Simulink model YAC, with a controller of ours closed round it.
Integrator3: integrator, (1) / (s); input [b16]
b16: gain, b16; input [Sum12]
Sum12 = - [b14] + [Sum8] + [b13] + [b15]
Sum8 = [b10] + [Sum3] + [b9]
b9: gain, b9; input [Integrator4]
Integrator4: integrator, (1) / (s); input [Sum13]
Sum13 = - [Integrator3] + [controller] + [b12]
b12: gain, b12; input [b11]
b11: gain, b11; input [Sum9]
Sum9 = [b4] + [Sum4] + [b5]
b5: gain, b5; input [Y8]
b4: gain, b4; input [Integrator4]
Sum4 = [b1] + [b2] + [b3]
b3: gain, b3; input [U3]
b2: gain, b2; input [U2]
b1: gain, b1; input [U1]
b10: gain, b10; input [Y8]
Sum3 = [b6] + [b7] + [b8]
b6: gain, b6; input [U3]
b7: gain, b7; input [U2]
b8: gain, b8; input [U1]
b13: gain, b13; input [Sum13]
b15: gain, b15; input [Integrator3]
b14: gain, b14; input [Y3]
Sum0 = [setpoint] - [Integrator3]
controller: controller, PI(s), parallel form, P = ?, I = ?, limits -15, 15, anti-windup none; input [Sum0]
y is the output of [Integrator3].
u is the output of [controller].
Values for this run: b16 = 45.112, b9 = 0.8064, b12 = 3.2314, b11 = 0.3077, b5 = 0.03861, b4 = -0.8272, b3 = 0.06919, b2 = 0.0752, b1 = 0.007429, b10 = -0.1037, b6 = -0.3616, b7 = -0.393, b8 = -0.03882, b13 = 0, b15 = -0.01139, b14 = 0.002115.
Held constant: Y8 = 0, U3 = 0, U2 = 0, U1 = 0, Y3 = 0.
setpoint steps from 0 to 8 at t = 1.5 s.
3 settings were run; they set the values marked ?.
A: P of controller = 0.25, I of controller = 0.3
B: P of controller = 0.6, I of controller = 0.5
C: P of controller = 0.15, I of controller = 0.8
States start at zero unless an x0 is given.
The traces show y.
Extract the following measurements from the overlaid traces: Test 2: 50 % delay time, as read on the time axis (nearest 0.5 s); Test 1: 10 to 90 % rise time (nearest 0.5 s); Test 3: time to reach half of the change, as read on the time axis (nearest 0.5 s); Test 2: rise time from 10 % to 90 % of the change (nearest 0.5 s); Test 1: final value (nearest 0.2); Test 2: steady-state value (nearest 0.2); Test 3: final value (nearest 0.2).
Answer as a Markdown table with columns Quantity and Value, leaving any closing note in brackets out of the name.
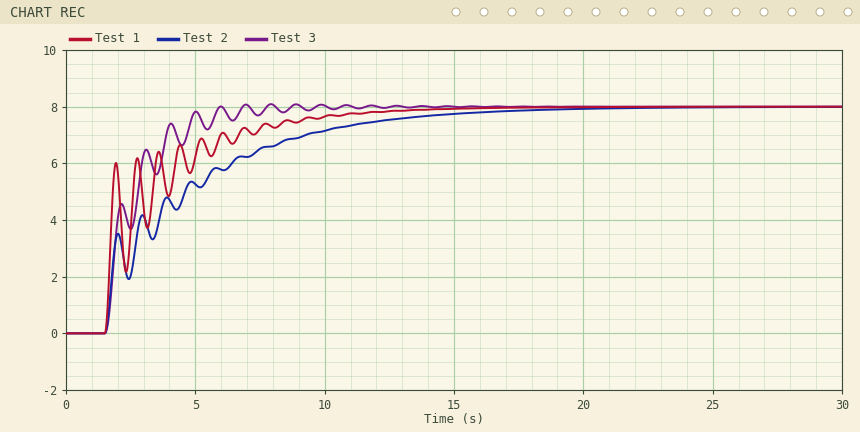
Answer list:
| Quantity | Value |
|---|---|
| Test 2: 50 % delay time, as read on the time axis | 3.0 s |
| Test 1: 10 to 90 % rise time | 5.0 s |
| Test 3: time to reach half of the change, as read on the time axis | 2.0 s |
| Test 2: rise time from 10 % to 90 % of the change | 8.5 s |
| Test 1: final value | 8.0 |
| Test 2: steady-state value | 8.0 |
| Test 3: final value | 8.0 |
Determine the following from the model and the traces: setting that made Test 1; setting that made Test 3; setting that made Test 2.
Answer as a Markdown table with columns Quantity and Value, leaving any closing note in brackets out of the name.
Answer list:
| Quantity | Value |
|---|---|
| setting that made Test 1 | B |
| setting that made Test 3 | C |
| setting that made Test 2 | A |
